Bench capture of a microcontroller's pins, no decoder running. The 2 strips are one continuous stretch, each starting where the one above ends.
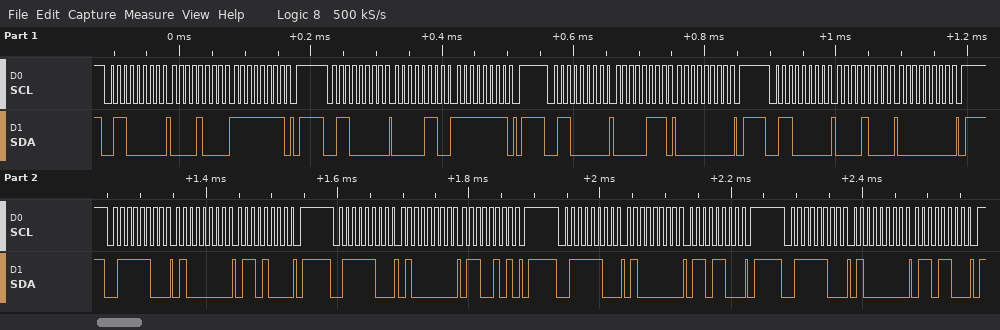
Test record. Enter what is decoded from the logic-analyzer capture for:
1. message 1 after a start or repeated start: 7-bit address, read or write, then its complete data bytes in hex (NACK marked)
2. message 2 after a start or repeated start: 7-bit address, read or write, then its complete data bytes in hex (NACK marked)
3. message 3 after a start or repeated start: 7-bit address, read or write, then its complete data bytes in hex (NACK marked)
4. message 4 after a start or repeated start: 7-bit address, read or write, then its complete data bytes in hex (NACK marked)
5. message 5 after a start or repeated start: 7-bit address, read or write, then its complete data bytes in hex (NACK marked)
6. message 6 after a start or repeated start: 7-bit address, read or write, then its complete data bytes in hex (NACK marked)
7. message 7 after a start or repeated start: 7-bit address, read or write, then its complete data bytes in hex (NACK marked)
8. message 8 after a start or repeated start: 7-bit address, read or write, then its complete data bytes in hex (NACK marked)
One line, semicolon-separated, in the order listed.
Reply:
0x30 write: 08 FF; 0x30 write: 06 FF; 0x30 write: 07 00; 0x30 write: 08 00; 0x3E write: 40 68; 0x3E write: 40 65; 0x3E write: 40 6C; 0x3E write: 40 6C
